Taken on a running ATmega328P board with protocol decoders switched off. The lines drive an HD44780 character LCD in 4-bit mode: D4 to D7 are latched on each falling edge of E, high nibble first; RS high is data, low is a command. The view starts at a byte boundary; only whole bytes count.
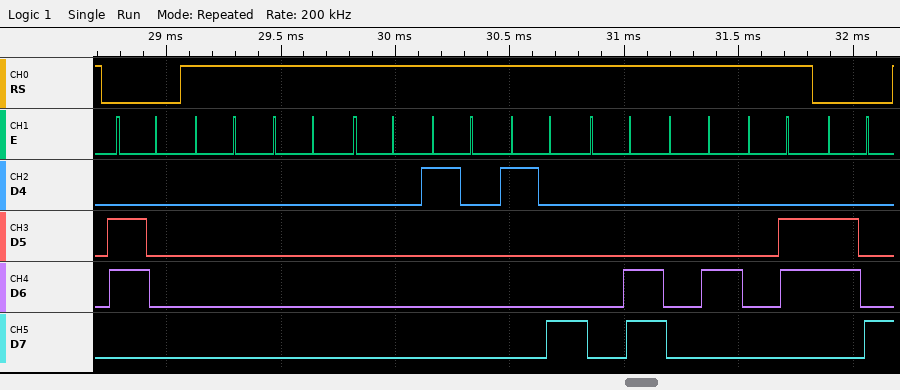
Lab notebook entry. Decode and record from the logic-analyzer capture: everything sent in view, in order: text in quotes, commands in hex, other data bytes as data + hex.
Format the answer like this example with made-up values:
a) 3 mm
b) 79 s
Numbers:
a) 0x60 data 00 00 00 10 18 0C 04 06 0x68
